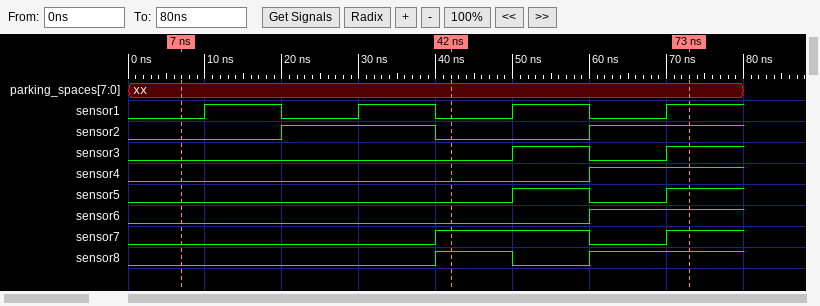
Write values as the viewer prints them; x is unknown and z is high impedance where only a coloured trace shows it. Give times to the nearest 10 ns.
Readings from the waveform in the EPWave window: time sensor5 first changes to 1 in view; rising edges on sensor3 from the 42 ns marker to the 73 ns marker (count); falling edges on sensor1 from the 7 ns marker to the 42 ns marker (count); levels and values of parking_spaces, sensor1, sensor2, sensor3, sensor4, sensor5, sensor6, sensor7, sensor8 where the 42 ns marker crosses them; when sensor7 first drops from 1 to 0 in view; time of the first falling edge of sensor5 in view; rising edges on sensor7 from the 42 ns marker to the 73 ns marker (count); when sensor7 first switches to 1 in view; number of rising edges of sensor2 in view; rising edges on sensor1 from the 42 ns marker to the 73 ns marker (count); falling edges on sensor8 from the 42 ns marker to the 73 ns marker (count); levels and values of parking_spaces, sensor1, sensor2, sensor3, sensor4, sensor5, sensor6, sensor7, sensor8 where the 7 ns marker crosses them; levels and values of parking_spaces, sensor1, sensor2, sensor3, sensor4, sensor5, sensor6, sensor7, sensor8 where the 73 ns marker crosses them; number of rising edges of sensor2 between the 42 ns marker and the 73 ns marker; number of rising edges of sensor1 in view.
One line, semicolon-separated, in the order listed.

50 ns; 2; 2; parking_spaces=xx, sensor1=0, sensor2=0, sensor3=0, sensor4=0, sensor5=0, sensor6=0, sensor7=1, sensor8=1; 60 ns; 60 ns; 1; 40 ns; 2; 2; 1; parking_spaces=xx, sensor1=0, sensor2=0, sensor3=0, sensor4=0, sensor5=0, sensor6=0, sensor7=0, sensor8=0; parking_spaces=xx, sensor1=1, sensor2=1, sensor3=1, sensor4=1, sensor5=1, sensor6=1, sensor7=1, sensor8=1; 1; 4
